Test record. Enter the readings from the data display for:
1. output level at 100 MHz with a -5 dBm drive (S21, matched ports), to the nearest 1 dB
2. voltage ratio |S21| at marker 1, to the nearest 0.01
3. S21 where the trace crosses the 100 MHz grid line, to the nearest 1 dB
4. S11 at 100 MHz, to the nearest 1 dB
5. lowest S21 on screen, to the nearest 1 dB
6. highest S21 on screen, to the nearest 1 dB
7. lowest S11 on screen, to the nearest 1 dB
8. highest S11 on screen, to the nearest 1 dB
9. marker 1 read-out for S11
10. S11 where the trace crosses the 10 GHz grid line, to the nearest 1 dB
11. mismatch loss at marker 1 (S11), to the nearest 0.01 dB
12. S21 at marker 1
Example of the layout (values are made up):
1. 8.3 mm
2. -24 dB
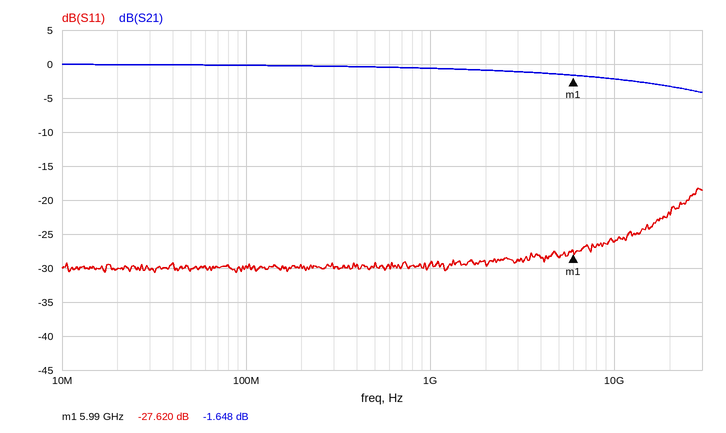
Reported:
1. -5 dBm
2. 0.83
3. 0 dB
4. -30 dB
5. -4 dB
6. 0 dB
7. -31 dB
8. -18 dB
9. -27.620 dB
10. -26 dB
11. 0.01 dB
12. -1.648 dB
